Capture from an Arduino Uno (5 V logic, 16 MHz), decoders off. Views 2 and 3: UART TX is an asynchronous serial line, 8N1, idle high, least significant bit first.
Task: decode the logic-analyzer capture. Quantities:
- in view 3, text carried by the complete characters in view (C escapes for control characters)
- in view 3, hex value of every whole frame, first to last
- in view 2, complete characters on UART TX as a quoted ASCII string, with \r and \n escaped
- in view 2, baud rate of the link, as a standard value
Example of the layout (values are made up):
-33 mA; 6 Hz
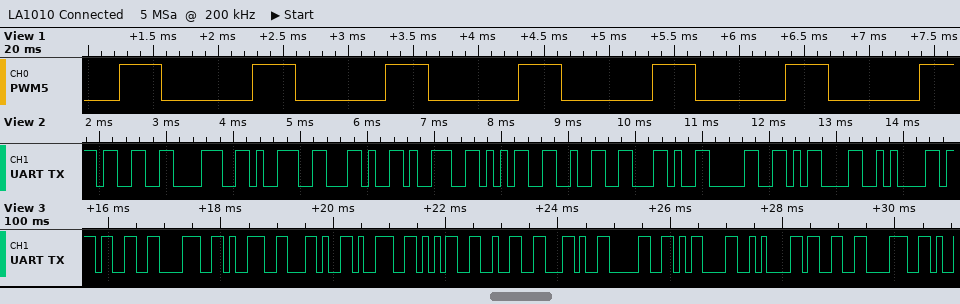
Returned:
"389,952,0\r\n38"; 33 38 39 2C 39 35 32 2C 30 0D 0A 33 38; "389,952,0\r\n"; 9600 baud
